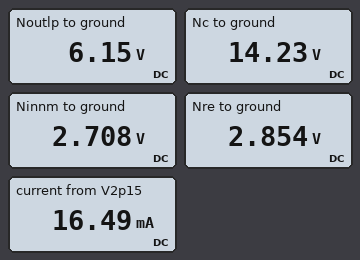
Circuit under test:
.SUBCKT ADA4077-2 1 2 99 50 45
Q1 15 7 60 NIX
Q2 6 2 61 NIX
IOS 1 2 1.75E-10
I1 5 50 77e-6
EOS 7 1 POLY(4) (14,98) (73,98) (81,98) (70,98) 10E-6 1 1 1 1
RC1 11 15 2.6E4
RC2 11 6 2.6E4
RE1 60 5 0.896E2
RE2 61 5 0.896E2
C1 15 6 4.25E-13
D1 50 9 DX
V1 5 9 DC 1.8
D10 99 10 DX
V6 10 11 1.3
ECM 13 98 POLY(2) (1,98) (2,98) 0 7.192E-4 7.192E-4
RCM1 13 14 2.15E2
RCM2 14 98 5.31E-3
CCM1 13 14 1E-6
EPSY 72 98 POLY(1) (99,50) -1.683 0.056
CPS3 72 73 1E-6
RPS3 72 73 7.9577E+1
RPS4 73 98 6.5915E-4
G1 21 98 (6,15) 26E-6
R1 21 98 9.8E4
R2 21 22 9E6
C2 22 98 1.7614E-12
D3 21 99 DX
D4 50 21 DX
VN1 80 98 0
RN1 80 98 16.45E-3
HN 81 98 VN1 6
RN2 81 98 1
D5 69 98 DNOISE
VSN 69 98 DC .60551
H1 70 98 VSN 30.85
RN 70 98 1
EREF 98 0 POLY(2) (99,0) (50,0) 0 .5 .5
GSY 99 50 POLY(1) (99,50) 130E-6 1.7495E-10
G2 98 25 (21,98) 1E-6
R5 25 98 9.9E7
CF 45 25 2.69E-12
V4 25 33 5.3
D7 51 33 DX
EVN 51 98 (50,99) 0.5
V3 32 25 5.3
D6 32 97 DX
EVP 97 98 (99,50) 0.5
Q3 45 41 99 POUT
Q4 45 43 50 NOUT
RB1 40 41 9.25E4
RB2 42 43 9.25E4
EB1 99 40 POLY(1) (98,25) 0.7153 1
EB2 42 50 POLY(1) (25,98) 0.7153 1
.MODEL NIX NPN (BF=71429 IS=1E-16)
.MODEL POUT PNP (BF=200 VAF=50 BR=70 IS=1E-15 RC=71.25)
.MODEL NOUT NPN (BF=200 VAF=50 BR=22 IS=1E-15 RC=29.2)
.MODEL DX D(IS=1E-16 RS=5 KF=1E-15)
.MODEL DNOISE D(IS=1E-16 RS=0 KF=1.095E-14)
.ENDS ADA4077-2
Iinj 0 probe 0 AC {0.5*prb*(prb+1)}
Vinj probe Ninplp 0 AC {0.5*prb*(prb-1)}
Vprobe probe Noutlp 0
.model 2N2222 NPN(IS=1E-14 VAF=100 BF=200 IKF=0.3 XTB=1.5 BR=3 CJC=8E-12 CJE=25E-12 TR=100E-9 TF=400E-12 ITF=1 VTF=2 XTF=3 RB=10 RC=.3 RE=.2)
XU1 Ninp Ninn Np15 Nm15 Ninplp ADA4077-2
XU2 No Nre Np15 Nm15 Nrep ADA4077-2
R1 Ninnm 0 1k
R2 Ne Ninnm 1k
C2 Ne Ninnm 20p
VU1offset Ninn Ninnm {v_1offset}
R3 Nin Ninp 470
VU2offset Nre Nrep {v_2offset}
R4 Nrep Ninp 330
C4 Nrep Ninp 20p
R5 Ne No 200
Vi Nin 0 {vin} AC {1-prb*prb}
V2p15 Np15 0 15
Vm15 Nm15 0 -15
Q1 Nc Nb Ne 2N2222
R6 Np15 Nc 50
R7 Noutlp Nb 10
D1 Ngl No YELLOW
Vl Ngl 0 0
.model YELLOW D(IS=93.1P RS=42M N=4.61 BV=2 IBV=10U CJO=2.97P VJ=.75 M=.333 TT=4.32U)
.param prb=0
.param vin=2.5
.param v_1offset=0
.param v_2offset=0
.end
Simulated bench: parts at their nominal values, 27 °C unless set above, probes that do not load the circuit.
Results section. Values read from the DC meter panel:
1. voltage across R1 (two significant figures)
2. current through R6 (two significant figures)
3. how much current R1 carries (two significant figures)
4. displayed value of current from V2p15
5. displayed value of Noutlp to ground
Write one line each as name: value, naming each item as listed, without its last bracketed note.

voltage across R1: 2.7 V
current through R6: 15 mA
how much current R1 carries: 2.7 mA
displayed value of current from V2p15: 16.49 mA
displayed value of Noutlp to ground: 6.15 V
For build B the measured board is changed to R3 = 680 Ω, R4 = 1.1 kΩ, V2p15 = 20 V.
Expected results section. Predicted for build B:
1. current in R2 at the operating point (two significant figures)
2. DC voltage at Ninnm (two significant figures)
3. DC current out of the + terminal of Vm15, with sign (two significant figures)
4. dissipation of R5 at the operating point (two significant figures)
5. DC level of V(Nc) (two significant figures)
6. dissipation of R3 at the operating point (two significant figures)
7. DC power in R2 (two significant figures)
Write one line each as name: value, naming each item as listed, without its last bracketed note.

current in R2 at the operating point: 2.6 mA
DC voltage at Ninnm: 2.6 V
DC current out of the + terminal of Vm15, with sign: -610 µA
dissipation of R5 at the operating point: 29 mW
DC level of V(Nc): 19 V
dissipation of R3 at the operating point: 26 µW
DC power in R2: 6.9 mW
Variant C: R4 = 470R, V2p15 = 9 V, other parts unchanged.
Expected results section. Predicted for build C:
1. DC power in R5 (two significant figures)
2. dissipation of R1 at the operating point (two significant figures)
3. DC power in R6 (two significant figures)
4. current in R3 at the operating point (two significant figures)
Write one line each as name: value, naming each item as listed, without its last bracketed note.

DC power in R5: 31 mW
dissipation of R1 at the operating point: 7.2 mW
DC power in R6: 11 mW
current in R3 at the operating point: 370 µA
